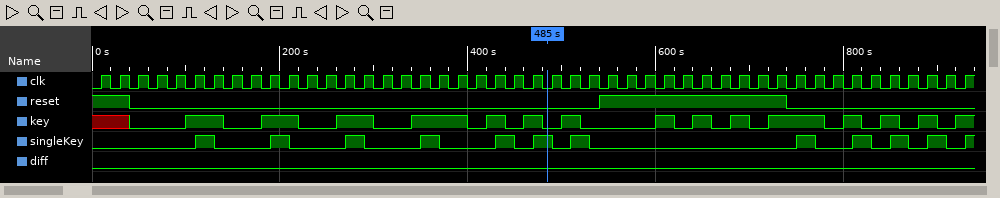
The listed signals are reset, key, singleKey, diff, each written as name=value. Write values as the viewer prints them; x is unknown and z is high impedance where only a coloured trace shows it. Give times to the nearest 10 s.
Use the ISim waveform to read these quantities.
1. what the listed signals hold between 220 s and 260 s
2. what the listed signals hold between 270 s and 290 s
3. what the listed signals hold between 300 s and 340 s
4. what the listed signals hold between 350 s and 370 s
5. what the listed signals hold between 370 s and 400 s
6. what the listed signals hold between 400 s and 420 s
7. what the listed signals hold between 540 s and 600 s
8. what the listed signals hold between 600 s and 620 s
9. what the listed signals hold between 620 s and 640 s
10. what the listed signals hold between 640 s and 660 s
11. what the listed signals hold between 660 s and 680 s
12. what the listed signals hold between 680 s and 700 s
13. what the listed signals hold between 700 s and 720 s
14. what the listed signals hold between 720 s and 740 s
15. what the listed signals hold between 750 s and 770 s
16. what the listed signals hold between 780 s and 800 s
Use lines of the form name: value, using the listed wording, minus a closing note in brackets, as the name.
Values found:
what the listed signals hold between 220 s and 260 s: reset=0, key=0, singleKey=0, diff=0
what the listed signals hold between 270 s and 290 s: reset=0, key=1, singleKey=1, diff=0
what the listed signals hold between 300 s and 340 s: reset=0, key=0, singleKey=0, diff=0
what the listed signals hold between 350 s and 370 s: reset=0, key=1, singleKey=1, diff=0
what the listed signals hold between 370 s and 400 s: reset=0, key=1, singleKey=0, diff=0
what the listed signals hold between 400 s and 420 s: reset=0, key=0, singleKey=0, diff=0
what the listed signals hold between 540 s and 600 s: reset=1, key=0, singleKey=0, diff=0
what the listed signals hold between 600 s and 620 s: reset=1, key=1, singleKey=0, diff=0
what the listed signals hold between 620 s and 640 s: reset=1, key=0, singleKey=0, diff=0
what the listed signals hold between 640 s and 660 s: reset=1, key=1, singleKey=0, diff=0
what the listed signals hold between 660 s and 680 s: reset=1, key=0, singleKey=0, diff=0
what the listed signals hold between 680 s and 700 s: reset=1, key=1, singleKey=0, diff=0
what the listed signals hold between 700 s and 720 s: reset=1, key=0, singleKey=0, diff=0
what the listed signals hold between 720 s and 740 s: reset=1, key=1, singleKey=0, diff=0
what the listed signals hold between 750 s and 770 s: reset=0, key=1, singleKey=1, diff=0
what the listed signals hold between 780 s and 800 s: reset=0, key=0, singleKey=0, diff=0
